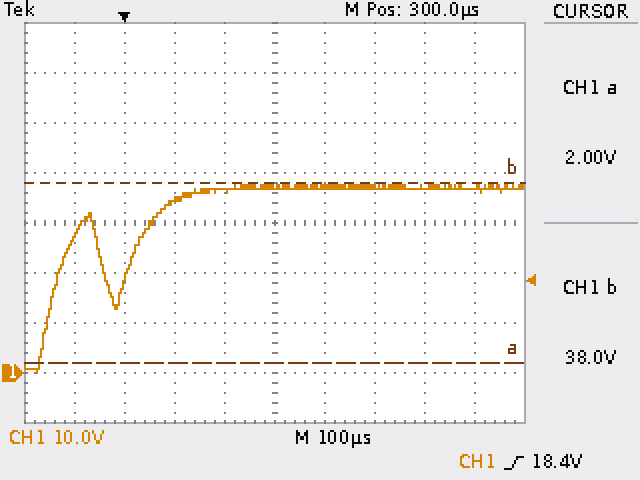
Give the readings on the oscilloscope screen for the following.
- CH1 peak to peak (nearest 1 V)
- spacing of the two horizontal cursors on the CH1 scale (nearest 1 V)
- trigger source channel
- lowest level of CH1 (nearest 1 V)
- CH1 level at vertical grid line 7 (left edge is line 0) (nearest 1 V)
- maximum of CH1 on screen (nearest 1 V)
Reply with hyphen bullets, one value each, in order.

- 38 V
- 36 V
- CH1
- 0 V
- 37 V
- 38 V
